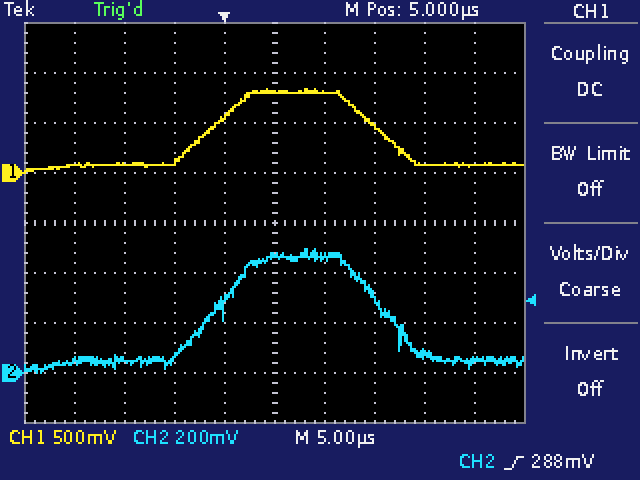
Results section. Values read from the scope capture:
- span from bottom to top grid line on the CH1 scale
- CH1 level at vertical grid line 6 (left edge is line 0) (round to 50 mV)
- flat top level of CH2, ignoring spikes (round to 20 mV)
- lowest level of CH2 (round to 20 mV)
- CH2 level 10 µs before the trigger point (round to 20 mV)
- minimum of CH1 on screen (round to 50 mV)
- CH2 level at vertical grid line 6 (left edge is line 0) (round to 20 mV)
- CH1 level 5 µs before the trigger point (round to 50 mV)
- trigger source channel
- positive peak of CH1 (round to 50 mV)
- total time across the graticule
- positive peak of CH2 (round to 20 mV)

4 V
800 mV
460 mV
0 mV
60 mV
0 mV
460 mV
100 mV
CH2
850 mV
50 µs
500 mV
